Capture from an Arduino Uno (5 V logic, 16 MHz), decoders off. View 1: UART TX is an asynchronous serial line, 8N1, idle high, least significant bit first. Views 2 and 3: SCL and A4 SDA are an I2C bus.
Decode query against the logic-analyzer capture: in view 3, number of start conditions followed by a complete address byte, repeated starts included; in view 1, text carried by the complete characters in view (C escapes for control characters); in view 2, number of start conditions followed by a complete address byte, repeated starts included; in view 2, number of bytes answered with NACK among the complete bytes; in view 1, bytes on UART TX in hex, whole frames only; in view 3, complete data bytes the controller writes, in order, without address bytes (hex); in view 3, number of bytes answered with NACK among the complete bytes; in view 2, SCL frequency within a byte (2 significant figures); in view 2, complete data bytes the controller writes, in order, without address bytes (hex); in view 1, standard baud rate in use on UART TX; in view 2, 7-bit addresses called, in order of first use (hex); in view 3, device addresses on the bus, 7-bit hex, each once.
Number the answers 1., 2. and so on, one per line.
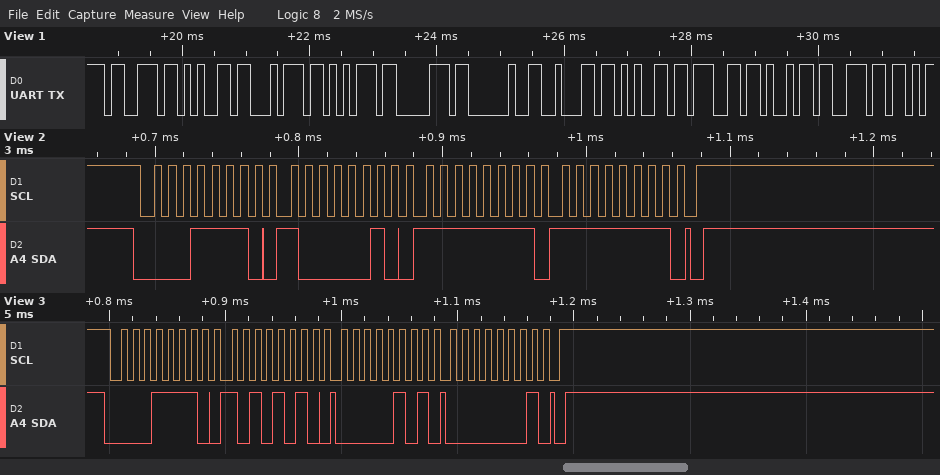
1. 1
2. "setup begin"
3. 1
4. 0
5. 73 65 74 75 70 20 62 65 67 69 6E
6. AA 05 01
7. 0
8. 100 kHz
9. 82 FF FF
10. 9600 baud
11. 0x0F
12. 0x0F
